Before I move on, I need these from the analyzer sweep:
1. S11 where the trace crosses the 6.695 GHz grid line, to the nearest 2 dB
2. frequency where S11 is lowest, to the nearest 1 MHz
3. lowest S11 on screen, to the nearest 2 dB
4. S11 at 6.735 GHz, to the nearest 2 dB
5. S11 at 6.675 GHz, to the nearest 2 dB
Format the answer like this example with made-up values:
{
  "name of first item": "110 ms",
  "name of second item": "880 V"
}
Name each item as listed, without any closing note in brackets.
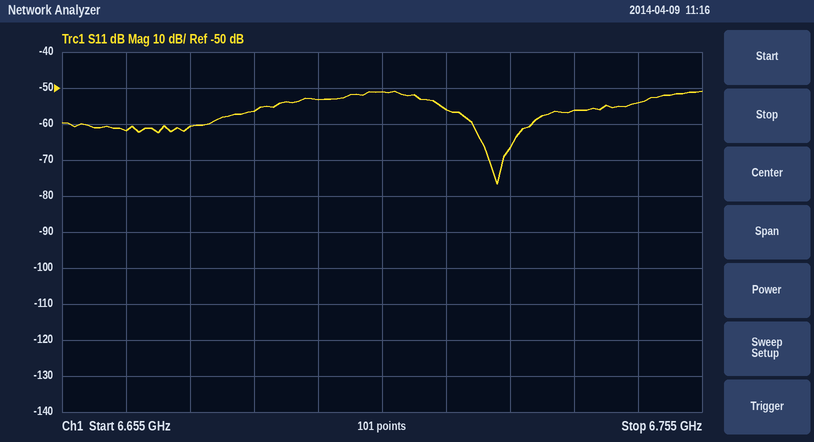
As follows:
{
  "S11 where the trace crosses the 6.695 GHz grid line, to the nearest 2 dB": "-54 dB",
  "frequency where S11 is lowest, to the nearest 1 MHz": "6.723 GHz",
  "lowest S11 on screen, to the nearest 2 dB": "-76 dB",
  "S11 at 6.735 GHz, to the nearest 2 dB": "-56 dB",
  "S11 at 6.675 GHz, to the nearest 2 dB": "-60 dB"
}
